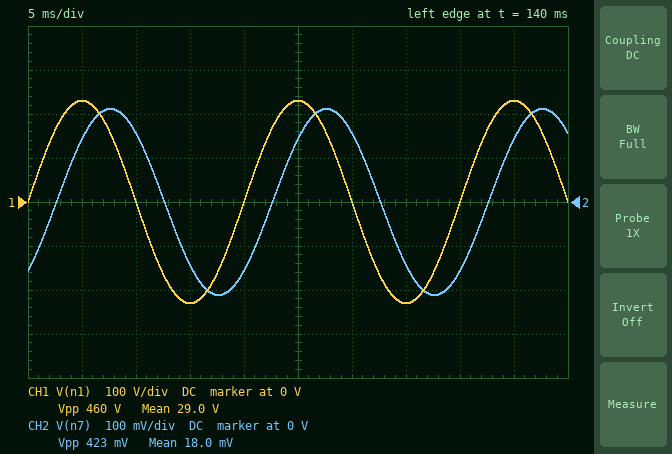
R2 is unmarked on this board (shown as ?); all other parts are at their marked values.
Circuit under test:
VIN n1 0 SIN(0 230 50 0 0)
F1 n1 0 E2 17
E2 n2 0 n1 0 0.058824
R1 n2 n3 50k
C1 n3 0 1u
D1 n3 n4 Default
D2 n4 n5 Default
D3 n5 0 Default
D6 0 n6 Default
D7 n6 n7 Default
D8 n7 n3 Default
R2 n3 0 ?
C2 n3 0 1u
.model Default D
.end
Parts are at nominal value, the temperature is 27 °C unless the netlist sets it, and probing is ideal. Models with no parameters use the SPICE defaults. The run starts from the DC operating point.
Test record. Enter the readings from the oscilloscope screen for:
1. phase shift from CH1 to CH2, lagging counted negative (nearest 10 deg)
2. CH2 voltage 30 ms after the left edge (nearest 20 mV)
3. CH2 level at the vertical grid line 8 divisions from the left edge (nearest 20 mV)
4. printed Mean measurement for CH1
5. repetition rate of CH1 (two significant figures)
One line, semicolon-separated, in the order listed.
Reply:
-50 deg; 160 mV; -160 mV; 29.0 V; 50 Hz
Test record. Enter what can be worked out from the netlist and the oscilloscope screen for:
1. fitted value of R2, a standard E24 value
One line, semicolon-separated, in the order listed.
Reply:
1.8 kΩ
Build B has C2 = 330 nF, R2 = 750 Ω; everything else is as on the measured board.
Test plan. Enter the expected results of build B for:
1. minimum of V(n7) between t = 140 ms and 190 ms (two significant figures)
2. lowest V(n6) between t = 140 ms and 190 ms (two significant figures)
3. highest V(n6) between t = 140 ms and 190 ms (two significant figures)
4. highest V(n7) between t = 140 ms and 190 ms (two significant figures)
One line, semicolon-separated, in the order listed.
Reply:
-130 mV; -64 mV; 64 mV; 130 mV
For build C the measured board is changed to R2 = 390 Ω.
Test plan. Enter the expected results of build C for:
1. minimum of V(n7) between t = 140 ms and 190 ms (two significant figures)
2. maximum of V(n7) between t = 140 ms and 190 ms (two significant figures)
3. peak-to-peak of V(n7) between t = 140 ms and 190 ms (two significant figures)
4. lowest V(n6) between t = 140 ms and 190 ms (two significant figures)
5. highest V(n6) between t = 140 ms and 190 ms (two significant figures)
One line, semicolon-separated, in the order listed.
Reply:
-68 mV; 68 mV; 140 mV; -34 mV; 34 mV
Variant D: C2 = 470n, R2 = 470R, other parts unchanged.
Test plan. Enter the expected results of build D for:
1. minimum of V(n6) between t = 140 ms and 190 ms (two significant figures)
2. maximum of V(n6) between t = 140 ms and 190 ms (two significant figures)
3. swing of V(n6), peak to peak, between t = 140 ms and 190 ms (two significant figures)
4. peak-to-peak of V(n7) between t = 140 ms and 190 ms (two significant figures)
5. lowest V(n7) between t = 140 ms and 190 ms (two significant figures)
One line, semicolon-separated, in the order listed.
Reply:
-41 mV; 41 mV; 82 mV; 160 mV; -82 mV
